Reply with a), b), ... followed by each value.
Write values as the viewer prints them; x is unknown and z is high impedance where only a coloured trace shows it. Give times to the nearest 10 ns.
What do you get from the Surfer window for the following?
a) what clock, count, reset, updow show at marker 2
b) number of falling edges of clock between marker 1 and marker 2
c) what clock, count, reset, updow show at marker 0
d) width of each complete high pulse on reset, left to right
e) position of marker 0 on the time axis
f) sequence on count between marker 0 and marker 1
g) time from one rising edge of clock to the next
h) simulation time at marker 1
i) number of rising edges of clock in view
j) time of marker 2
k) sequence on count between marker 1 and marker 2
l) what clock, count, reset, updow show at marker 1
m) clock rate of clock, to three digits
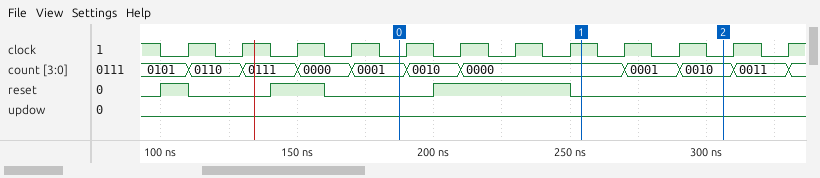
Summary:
a) clock=0, count=0010, reset=0, updow=0
b) 3
c) clock=0, count=0001, reset=0, updow=0
d) 10 ns, 20 ns, 50 ns
e) 190 ns
f) 0001, 0010, 0000
g) 20 ns
h) 250 ns
i) 12
j) 310 ns
k) 0000, 0001, 0010
l) clock=1, count=0000, reset=0, updow=0
m) 50.0 MHz
